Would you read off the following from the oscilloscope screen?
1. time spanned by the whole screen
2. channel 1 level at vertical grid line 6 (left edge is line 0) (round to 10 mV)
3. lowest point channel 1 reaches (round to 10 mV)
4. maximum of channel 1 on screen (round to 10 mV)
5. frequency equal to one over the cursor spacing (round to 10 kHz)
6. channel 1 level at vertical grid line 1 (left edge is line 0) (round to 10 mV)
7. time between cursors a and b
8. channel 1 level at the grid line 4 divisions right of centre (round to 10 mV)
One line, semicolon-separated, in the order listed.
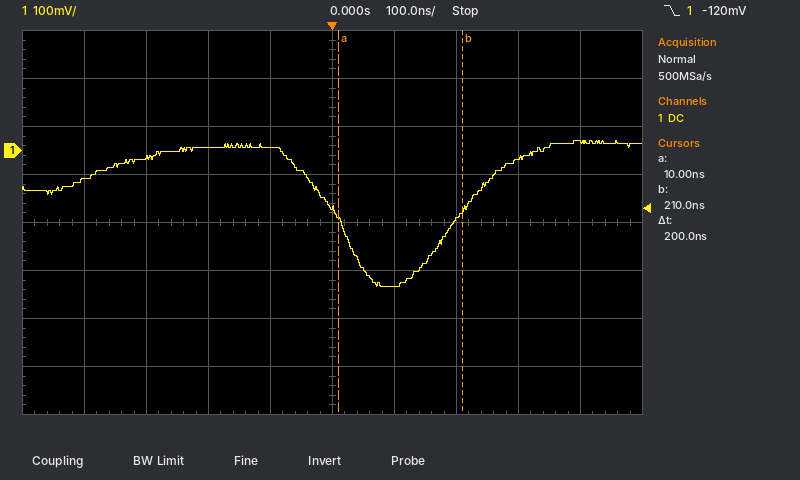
1 µs; -280 mV; -280 mV; 20 mV; 5.00 MHz; -60 mV; 200 ns; 20 mV
